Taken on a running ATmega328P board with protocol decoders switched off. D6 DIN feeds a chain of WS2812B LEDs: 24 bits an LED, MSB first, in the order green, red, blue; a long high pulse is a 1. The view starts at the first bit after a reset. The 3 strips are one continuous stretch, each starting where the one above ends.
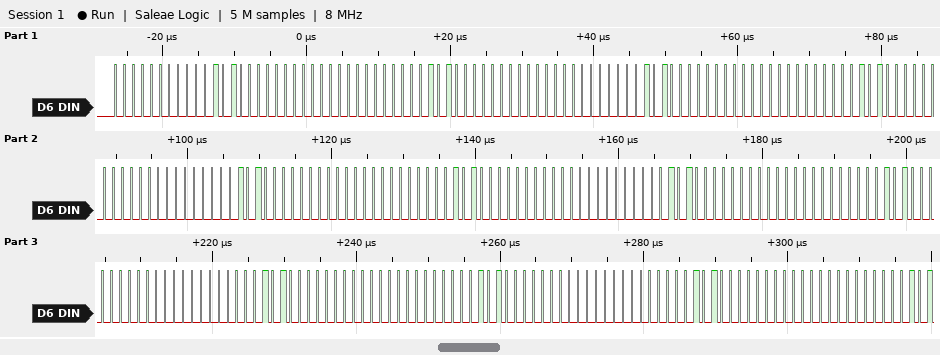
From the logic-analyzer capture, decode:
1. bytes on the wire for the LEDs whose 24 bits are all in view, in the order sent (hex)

00 14 00 00 14 00 00 14 00 00 14 00 00 14 00 00 14 00 00 14 00 00 14 00 00 14 00 00 14 00 00 14 00
